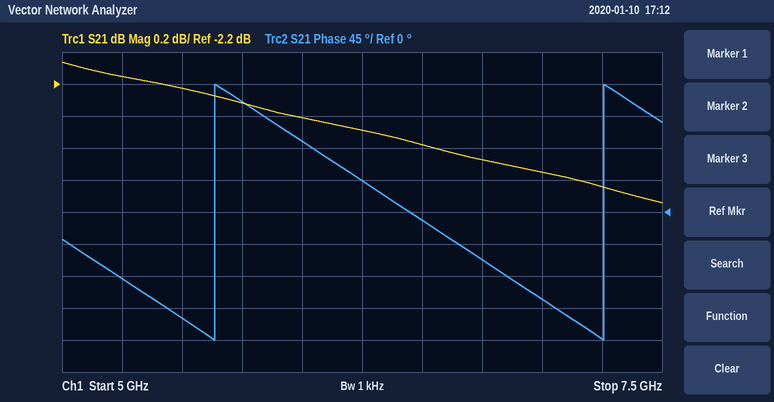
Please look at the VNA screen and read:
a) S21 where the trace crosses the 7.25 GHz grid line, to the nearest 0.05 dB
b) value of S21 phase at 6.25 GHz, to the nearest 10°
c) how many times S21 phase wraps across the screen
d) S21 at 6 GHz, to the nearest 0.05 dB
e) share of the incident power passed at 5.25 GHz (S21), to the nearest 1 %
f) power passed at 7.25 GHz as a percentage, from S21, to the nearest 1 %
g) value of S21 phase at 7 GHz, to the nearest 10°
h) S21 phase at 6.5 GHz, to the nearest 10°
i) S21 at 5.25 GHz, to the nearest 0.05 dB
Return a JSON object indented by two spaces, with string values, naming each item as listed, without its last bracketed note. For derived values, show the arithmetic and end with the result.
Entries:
{
  "S21 where the trace crosses the 7.25 GHz grid line, to the nearest 0.05 dB": "-2.85 dB",
  "value of S21 phase at 6.25 GHz, to the nearest 10°": "40°",
  "how many times S21 phase wraps across the screen": "2",
  "S21 at 6 GHz, to the nearest 0.05 dB": "-2.40 dB",
  "share of the incident power passed at 5.25 GHz (S21), to the nearest 1 %": "10^(-2.15/10) ≈ 61 %",
  "power passed at 7.25 GHz as a percentage, from S21, to the nearest 1 %": "10^(-2.85/10) ≈ 52 %",
  "value of S21 phase at 7 GHz, to the nearest 10°": "-120°",
  "S21 phase at 6.5 GHz, to the nearest 10°": "-10°",
  "S21 at 5.25 GHz, to the nearest 0.05 dB": "-2.15 dB"
}
